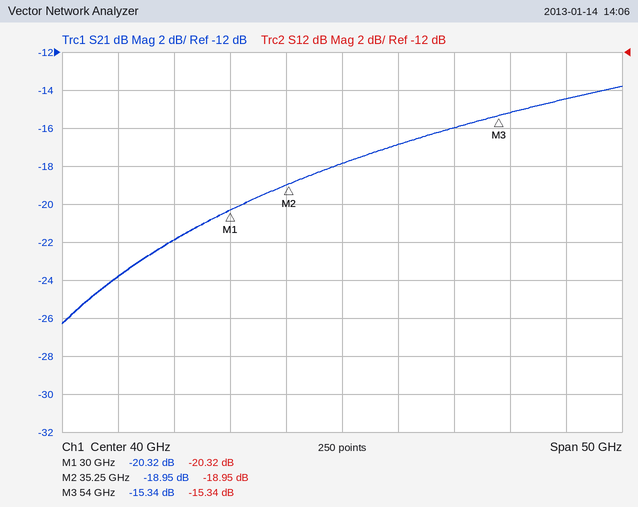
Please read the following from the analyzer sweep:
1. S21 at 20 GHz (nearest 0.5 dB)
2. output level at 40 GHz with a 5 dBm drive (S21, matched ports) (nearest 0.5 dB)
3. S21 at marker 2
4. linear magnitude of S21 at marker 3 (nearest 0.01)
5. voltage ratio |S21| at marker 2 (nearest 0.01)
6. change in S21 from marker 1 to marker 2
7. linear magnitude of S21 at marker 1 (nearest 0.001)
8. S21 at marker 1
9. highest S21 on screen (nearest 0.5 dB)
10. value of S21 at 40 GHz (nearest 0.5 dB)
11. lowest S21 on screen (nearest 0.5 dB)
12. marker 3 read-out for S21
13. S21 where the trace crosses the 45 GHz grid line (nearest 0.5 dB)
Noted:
-24.0 dB
-13.0 dBm
-18.95 dB
0.17
0.11
1.37 dB
0.096
-20.32 dB
-14.0 dB
-18.0 dB
-26.5 dB
-15.34 dB
-17.0 dB
